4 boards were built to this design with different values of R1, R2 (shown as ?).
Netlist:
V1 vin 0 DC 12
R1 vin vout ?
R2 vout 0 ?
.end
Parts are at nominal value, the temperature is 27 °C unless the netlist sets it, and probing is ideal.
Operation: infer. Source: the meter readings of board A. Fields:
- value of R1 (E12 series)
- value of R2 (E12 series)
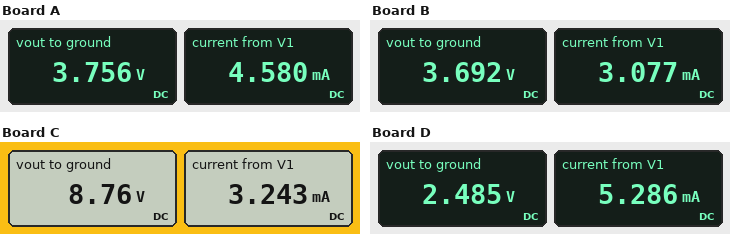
1.8 kΩ
820 Ω
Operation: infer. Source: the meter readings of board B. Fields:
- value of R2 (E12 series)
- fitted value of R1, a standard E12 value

1.2 kΩ
2.7 kΩ
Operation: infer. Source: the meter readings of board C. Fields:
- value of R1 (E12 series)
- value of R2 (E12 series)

1 kΩ
2.7 kΩ
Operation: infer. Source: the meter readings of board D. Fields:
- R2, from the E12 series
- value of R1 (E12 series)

470 Ω
1.8 kΩ
